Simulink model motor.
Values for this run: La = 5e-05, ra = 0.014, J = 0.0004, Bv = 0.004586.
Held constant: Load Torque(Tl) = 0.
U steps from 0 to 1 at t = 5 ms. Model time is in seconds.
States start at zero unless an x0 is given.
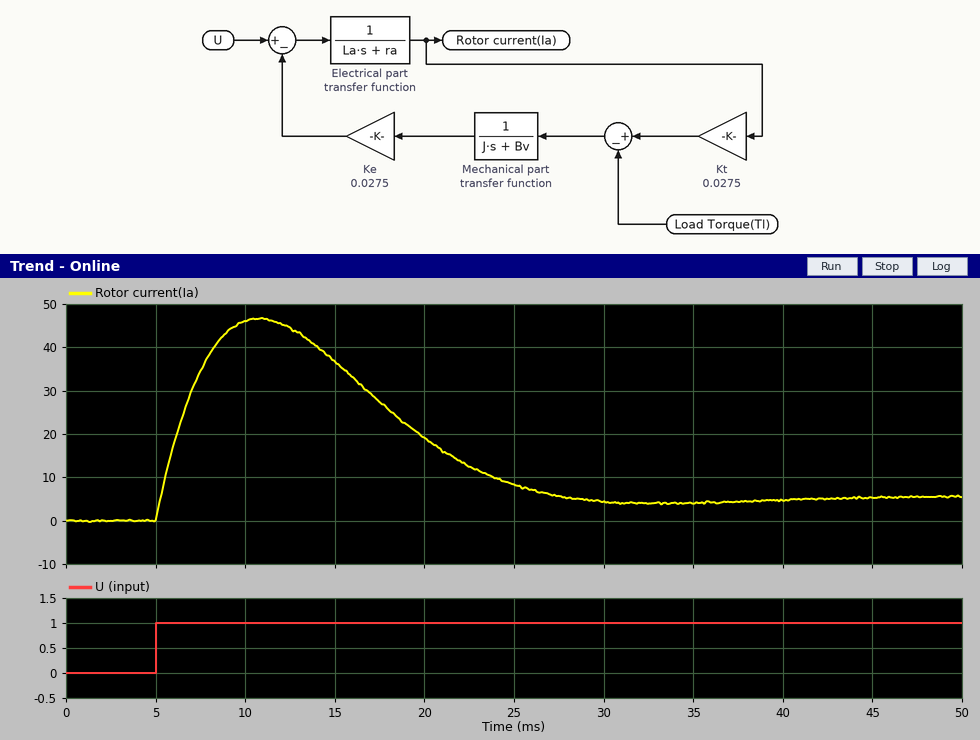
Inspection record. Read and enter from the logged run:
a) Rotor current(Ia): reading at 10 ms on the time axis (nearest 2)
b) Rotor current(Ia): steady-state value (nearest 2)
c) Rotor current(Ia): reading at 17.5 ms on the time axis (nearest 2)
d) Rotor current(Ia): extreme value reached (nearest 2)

46
6
28
46
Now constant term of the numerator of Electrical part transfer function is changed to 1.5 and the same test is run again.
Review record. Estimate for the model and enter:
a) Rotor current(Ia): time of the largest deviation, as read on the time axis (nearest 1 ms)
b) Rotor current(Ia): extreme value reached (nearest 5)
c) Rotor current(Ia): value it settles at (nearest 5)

10 ms
65
5
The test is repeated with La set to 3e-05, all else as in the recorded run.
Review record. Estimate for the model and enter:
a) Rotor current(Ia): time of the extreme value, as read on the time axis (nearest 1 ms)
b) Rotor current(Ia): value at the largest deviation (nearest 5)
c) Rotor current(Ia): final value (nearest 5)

9 ms
50
5
